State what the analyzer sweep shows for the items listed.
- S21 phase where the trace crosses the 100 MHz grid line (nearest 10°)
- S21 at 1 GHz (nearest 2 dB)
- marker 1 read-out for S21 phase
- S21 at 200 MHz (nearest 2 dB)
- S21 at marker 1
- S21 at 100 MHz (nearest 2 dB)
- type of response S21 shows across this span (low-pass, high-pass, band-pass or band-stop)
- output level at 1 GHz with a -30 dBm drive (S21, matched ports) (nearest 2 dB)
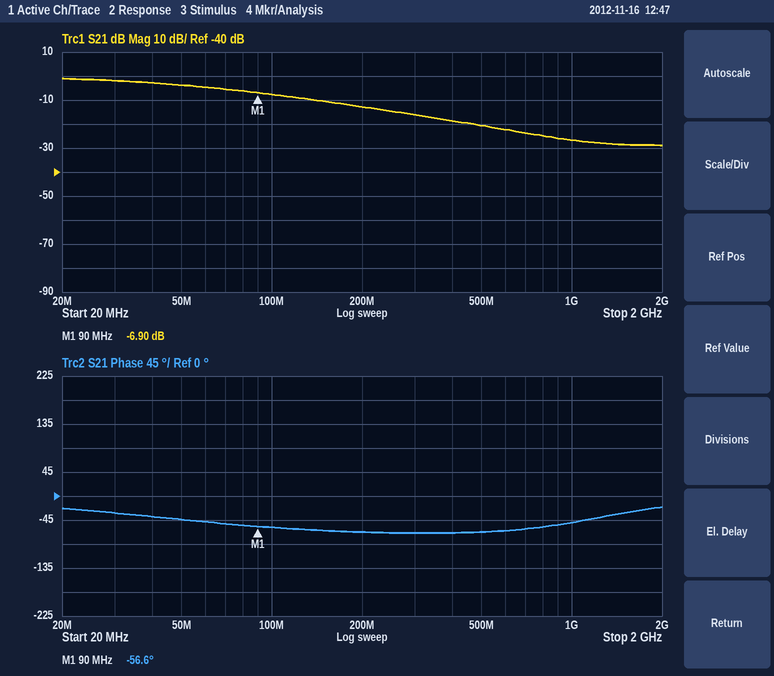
-60°
-26 dB
-56.6°
-12 dB
-6.90 dB
-8 dB
low-pass
-56 dBm
